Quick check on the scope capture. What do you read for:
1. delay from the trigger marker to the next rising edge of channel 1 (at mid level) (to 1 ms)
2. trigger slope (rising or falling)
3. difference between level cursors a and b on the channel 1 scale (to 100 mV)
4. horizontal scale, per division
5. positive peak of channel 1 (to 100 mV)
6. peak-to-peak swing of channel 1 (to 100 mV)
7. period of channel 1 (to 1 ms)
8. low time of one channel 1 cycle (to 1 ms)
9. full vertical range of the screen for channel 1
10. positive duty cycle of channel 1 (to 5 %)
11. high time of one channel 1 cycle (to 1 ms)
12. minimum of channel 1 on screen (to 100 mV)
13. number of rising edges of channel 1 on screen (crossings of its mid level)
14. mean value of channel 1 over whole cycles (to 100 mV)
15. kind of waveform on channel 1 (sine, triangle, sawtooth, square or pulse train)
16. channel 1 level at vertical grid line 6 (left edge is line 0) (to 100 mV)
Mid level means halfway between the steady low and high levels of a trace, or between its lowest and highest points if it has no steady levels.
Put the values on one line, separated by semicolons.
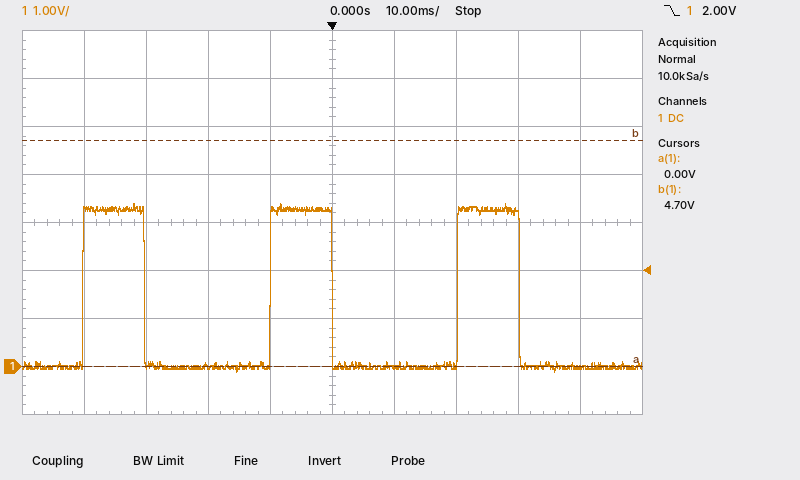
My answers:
20 ms; falling; 4.7 V; 10 ms; 3.4 V; 3.5 V; 30 ms; 20 ms; 8 V; 35 %; 10 ms; -100 mV; 3; 1.1 V; pulse train; 0.0 V
